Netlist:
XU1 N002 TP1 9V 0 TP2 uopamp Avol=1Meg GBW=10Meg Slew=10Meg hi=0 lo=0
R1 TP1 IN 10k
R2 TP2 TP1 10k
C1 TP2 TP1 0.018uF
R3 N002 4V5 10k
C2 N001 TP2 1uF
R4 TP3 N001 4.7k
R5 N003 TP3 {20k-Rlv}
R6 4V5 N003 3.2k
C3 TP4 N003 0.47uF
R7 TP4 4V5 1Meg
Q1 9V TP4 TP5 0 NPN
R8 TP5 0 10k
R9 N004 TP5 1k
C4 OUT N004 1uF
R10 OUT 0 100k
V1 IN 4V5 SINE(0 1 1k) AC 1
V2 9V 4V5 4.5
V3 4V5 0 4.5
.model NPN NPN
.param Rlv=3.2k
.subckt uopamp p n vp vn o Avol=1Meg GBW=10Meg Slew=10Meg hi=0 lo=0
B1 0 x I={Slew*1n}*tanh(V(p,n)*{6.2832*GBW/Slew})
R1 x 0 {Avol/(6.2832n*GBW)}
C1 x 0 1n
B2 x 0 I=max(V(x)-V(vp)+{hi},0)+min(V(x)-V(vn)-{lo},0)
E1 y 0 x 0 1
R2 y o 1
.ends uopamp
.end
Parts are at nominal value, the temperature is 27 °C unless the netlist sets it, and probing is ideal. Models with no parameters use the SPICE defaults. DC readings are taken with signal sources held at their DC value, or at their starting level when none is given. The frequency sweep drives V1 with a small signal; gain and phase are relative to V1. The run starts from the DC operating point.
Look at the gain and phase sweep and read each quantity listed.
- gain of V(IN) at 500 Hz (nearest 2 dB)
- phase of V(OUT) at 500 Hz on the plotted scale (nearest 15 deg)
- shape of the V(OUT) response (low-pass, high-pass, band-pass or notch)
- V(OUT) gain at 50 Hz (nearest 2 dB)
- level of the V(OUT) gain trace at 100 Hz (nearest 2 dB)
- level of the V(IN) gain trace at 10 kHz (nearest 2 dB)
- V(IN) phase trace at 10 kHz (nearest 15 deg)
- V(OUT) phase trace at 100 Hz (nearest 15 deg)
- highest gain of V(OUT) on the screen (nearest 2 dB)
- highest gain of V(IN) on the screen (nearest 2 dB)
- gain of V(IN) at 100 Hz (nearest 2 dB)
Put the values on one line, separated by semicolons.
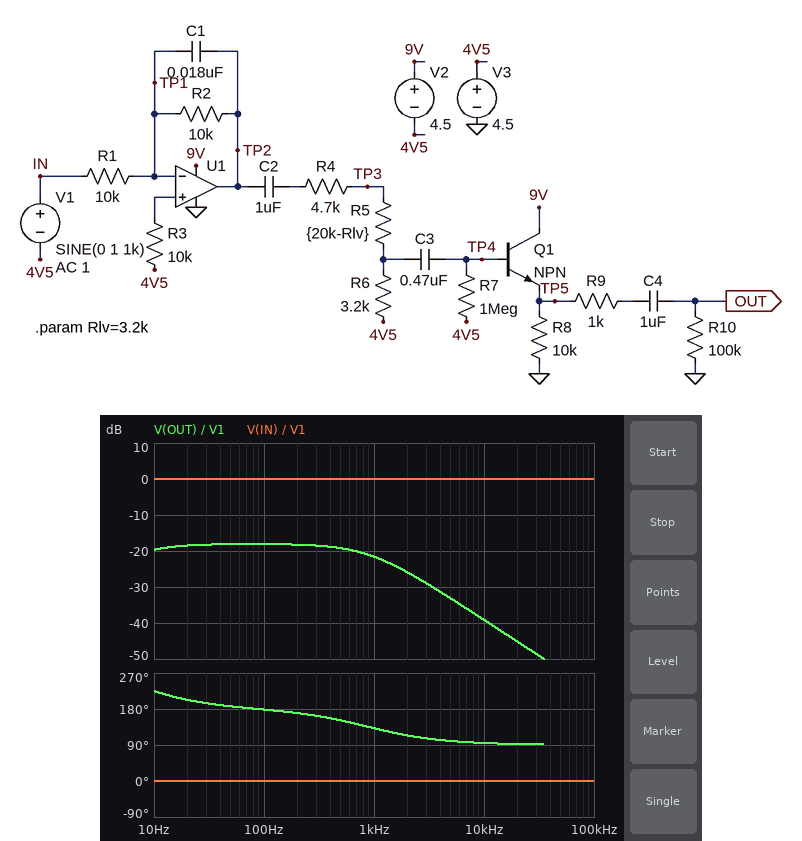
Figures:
0 dB; 150 deg; low-pass; -18 dB; -18 dB; 0 dB; 0 deg; 180 deg; -18 dB; 0 dB; 0 dB
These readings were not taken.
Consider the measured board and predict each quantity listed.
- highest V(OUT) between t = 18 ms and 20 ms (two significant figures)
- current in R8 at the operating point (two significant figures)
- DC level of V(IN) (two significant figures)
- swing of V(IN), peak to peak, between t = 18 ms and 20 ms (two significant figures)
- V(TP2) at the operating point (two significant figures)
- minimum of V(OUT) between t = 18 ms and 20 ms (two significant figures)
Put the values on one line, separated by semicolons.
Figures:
84 mV; 190 µA; 4.5 V; 2.0 V; 4.5 V; -83 mV
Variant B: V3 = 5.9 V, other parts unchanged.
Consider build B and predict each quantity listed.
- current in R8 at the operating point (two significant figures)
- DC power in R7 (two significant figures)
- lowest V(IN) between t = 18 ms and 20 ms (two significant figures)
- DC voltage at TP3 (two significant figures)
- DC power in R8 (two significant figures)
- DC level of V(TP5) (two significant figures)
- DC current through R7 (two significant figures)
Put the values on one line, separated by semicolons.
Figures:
260 µA; 6.6 µW; 4.9 V; 5.9 V; 670 µW; 2.6 V; 2.6 µA
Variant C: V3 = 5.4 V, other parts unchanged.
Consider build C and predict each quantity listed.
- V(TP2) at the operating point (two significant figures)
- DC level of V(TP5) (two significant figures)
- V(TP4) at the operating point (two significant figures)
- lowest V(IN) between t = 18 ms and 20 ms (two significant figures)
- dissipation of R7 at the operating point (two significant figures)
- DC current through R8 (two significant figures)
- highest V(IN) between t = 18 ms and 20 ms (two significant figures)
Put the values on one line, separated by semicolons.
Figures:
5.4 V; 2.3 V; 3.1 V; 4.4 V; 5.4 µW; 230 µA; 6.4 V
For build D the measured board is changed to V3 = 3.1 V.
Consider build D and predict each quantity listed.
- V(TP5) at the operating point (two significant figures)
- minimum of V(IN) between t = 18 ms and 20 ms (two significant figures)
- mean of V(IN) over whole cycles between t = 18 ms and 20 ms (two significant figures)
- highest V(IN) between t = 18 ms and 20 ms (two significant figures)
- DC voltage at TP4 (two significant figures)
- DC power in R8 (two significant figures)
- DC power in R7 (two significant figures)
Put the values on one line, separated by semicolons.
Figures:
1.2 V; 2.1 V; 3.1 V; 4.1 V; 1.9 V; 140 µW; 1.4 µW
